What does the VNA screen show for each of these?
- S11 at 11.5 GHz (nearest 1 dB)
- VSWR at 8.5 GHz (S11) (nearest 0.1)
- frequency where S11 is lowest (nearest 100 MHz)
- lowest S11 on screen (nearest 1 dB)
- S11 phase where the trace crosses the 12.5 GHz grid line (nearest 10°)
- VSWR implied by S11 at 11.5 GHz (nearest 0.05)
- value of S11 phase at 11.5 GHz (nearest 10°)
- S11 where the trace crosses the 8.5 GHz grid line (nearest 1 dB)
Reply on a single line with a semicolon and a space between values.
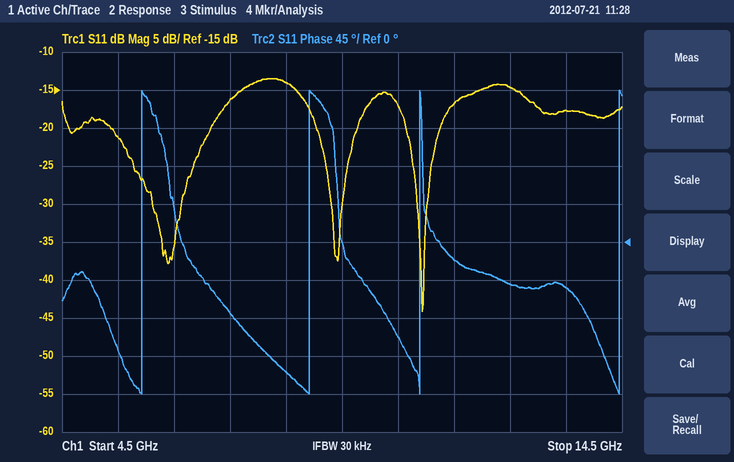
-17 dB; 1.5; 10.9 GHz; -44 dB; -50°; 1.35; -20°; -14 dB
